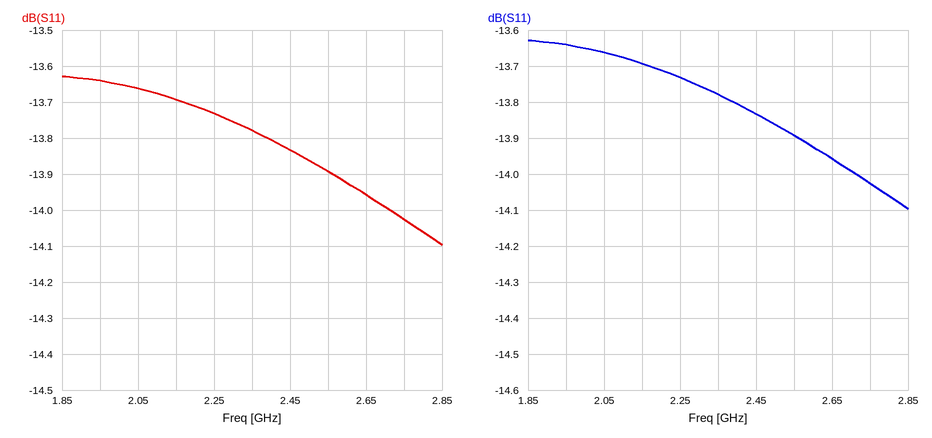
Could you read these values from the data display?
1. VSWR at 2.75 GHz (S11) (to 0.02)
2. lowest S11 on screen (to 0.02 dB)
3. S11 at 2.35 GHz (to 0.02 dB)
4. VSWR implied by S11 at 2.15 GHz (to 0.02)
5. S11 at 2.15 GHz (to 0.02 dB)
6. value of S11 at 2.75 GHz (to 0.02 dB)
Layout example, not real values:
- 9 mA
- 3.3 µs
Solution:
- 1.50
- -14.10 dB
- -13.78 dB
- 1.52
- -13.70 dB
- -14.02 dB
